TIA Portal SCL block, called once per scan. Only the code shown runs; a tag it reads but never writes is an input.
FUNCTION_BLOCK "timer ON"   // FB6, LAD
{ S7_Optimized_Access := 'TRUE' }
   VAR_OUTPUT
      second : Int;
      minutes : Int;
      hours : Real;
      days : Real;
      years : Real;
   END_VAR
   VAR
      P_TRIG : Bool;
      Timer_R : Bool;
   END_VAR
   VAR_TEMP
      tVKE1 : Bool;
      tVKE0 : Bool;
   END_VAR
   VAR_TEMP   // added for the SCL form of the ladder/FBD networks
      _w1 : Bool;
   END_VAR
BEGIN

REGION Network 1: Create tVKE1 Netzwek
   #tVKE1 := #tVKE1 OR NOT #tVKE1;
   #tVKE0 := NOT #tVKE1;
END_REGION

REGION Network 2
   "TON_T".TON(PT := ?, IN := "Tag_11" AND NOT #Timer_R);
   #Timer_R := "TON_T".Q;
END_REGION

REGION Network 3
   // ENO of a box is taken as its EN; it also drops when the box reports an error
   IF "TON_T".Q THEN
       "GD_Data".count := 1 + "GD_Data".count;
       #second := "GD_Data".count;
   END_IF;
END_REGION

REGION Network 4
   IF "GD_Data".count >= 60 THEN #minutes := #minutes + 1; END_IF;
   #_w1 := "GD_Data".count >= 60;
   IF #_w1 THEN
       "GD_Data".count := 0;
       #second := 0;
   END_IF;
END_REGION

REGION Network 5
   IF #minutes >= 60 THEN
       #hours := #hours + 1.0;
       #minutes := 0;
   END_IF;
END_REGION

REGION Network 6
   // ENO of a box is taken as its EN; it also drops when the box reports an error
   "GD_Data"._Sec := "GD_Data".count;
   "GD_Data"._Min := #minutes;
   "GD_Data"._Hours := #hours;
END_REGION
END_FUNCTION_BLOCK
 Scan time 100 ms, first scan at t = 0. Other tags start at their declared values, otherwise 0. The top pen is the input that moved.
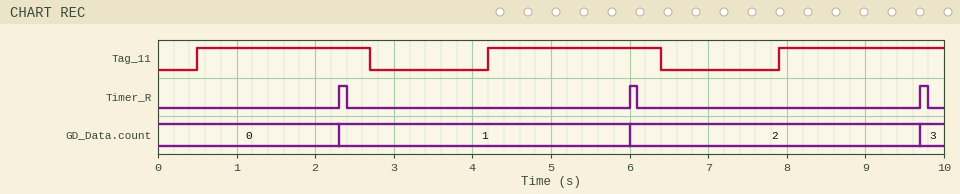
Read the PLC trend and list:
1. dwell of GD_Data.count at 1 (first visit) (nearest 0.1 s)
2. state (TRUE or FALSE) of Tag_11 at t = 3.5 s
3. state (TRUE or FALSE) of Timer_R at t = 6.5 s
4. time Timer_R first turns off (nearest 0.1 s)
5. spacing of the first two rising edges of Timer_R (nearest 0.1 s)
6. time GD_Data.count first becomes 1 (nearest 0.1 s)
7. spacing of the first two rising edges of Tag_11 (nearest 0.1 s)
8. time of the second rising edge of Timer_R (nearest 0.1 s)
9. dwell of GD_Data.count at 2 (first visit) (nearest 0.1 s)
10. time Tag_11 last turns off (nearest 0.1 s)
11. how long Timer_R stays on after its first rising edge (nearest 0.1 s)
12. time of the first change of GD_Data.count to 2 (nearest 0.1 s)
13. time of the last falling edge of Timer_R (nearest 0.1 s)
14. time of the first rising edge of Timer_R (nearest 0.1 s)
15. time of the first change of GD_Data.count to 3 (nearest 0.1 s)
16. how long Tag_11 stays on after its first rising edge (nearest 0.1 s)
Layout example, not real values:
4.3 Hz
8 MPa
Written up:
3.7 s
FALSE
FALSE
2.4 s
3.7 s
2.3 s
3.7 s
6.0 s
3.7 s
6.4 s
0.1 s
6.0 s
9.8 s
2.3 s
9.7 s
2.2 s
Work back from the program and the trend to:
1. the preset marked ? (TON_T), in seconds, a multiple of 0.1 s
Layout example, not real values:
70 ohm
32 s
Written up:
1.8 s
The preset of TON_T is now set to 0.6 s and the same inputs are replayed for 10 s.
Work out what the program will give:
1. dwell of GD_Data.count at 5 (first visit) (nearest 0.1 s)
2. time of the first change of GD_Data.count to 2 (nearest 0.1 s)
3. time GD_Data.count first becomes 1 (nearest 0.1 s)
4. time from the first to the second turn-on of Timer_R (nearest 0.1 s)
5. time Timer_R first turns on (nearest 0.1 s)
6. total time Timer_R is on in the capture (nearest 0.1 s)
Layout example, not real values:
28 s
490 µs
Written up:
0.8 s
1.9 s
1.1 s
0.8 s
1.1 s
0.6 s
